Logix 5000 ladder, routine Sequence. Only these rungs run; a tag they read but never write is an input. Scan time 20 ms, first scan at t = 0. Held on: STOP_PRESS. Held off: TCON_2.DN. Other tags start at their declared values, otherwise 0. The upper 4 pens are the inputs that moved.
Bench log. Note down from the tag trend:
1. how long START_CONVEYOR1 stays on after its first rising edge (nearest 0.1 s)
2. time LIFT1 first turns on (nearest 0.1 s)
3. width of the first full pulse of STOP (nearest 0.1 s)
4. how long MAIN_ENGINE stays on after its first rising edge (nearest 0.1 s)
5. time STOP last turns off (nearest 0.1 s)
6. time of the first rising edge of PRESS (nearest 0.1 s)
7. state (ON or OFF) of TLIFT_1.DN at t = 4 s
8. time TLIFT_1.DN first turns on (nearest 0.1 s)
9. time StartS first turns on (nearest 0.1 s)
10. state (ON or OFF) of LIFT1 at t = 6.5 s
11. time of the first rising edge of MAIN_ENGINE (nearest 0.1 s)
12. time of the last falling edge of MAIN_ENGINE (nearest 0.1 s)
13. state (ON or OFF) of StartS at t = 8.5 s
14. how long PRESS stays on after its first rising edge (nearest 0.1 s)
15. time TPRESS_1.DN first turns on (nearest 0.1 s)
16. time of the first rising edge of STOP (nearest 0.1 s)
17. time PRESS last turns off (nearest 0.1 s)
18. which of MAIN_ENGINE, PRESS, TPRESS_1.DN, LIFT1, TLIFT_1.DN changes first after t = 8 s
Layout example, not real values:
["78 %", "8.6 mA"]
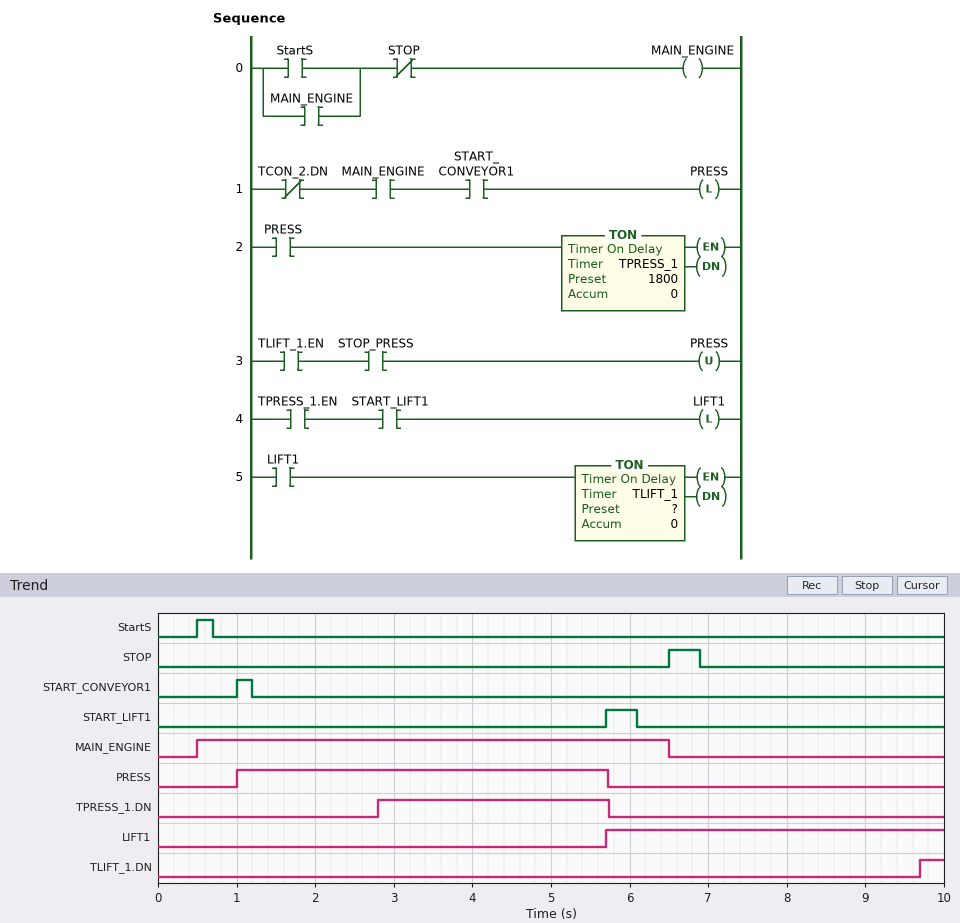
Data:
["0.2 s", "5.7 s", "0.4 s", "6.0 s", "6.9 s", "1.0 s", "OFF", "9.7 s", "0.5 s", "ON", "0.5 s", "6.5 s", "OFF", "4.7 s", "2.8 s", "6.5 s", "5.7 s", "TLIFT_1.DN"]
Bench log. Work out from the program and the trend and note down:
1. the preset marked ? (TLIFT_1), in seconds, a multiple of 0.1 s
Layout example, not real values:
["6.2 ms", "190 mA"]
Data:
["4.0 s"]
